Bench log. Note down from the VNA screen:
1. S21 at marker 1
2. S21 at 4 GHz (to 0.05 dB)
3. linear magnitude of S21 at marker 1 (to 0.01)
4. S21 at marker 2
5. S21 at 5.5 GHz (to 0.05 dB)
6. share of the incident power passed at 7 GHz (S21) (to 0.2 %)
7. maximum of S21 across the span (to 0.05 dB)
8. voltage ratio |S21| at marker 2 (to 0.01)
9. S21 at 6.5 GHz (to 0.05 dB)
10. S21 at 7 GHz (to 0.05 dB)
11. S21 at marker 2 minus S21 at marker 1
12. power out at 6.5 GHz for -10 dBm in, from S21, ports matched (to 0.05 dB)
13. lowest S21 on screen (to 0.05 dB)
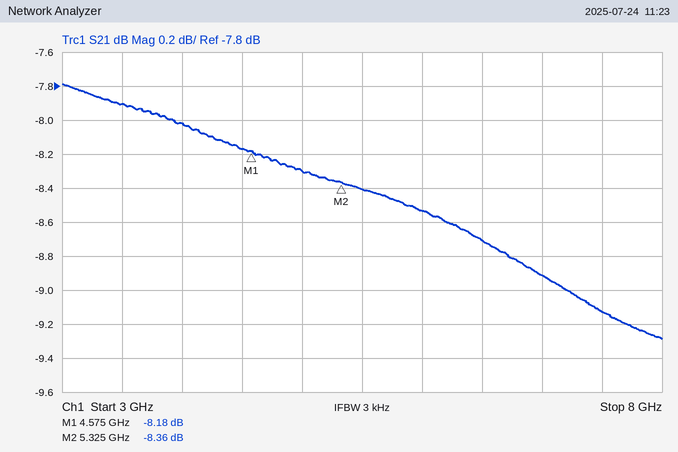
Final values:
-8.18 dB
-8.00 dB
0.39
-8.36 dB
-8.40 dB
12.8 %
-7.80 dB
0.38
-8.70 dB
-8.90 dB
-0.18 dB
-18.70 dBm
-9.30 dB
